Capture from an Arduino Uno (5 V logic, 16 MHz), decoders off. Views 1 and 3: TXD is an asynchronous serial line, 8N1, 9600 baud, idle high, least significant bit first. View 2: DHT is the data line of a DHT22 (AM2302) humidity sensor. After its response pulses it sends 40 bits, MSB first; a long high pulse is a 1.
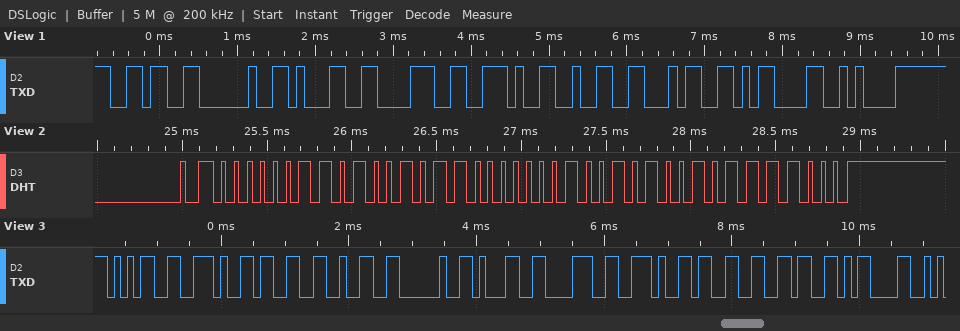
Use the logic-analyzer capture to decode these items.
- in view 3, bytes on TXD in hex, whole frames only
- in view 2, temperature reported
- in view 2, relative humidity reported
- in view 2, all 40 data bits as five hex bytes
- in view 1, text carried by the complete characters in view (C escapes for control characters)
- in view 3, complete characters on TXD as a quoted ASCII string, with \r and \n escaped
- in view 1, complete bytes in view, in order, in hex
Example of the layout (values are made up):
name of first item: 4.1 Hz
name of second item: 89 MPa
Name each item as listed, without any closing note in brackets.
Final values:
in view 3, bytes on TXD in hex, whole frames only: 0x35 0x2E 0x33 0x32 0x20 0x31 0x38 0x2E 0x33 0x36 0x0D
in view 2, temperature reported: 29.7 °C
in view 2, relative humidity reported: 84.3 %
in view 2, all 40 data bits as five hex bytes: 03 4B 01 29 78
in view 1, text carried by the complete characters in view: "6 18.24\r\n"
in view 3, complete characters on TXD as a quoted ASCII string, with \r and \n escaped: "5.32 18.36\r"
in view 1, complete bytes in view, in order, in hex: 36 20 31 38 2E 32 34 0D 0A
